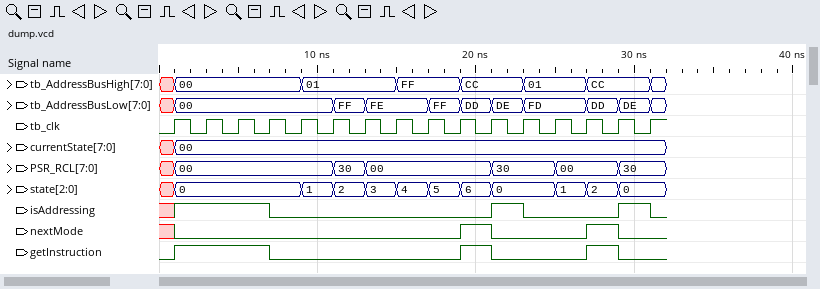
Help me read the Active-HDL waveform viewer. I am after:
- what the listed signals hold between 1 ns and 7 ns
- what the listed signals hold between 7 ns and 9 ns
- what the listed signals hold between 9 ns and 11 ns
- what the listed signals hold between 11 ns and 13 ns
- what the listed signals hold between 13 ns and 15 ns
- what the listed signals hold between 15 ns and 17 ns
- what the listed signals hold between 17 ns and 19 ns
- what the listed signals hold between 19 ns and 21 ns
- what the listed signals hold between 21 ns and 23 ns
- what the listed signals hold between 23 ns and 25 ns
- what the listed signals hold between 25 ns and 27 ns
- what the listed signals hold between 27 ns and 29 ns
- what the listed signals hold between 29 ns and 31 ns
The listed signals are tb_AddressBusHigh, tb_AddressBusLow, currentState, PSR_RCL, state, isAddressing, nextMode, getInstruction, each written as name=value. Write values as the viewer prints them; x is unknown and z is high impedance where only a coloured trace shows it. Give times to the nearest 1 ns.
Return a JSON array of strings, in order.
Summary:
["tb_AddressBusHigh=00, tb_AddressBusLow=00, currentState=00, PSR_RCL=00, state=0, isAddressing=1, nextMode=0, getInstruction=1", "tb_AddressBusHigh=00, tb_AddressBusLow=00, currentState=00, PSR_RCL=00, state=0, isAddressing=0, nextMode=0, getInstruction=0", "tb_AddressBusHigh=01, tb_AddressBusLow=00, currentState=00, PSR_RCL=00, state=1, isAddressing=0, nextMode=0, getInstruction=0", "tb_AddressBusHigh=01, tb_AddressBusLow=FF, currentState=00, PSR_RCL=30, state=2, isAddressing=0, nextMode=0, getInstruction=0", "tb_AddressBusHigh=01, tb_AddressBusLow=FE, currentState=00, PSR_RCL=00, state=3, isAddressing=0, nextMode=0, getInstruction=0", "tb_AddressBusHigh=FF, tb_AddressBusLow=FE, currentState=00, PSR_RCL=00, state=4, isAddressing=0, nextMode=0, getInstruction=0", "tb_AddressBusHigh=FF, tb_AddressBusLow=FF, currentState=00, PSR_RCL=00, state=5, isAddressing=0, nextMode=0, getInstruction=0", "tb_AddressBusHigh=CC, tb_AddressBusLow=DD, currentState=00, PSR_RCL=00, state=6, isAddressing=0, nextMode=1, getInstruction=1", "tb_AddressBusHigh=CC, tb_AddressBusLow=DE, currentState=00, PSR_RCL=30, state=0, isAddressing=1, nextMode=0, getInstruction=0", "tb_AddressBusHigh=01, tb_AddressBusLow=FD, currentState=00, PSR_RCL=30, state=0, isAddressing=0, nextMode=0, getInstruction=0", "tb_AddressBusHigh=01, tb_AddressBusLow=FD, currentState=00, PSR_RCL=00, state=1, isAddressing=0, nextMode=0, getInstruction=0", "tb_AddressBusHigh=CC, tb_AddressBusLow=DD, currentState=00, PSR_RCL=00, state=2, isAddressing=0, nextMode=1, getInstruction=1", "tb_AddressBusHigh=CC, tb_AddressBusLow=DE, currentState=00, PSR_RCL=30, state=0, isAddressing=1, nextMode=0, getInstruction=0"]
